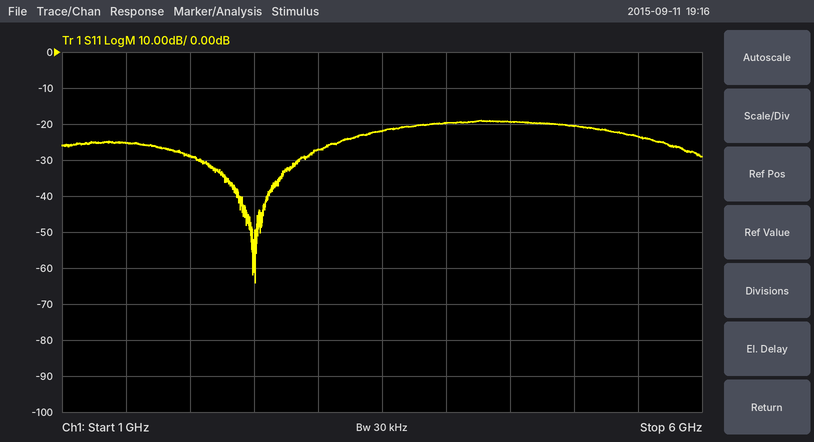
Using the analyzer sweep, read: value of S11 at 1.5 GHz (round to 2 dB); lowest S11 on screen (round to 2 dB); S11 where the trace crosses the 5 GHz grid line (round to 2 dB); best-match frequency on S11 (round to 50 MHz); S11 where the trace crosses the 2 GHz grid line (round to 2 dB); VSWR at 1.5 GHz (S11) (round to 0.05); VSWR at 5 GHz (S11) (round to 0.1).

-26 dB
-64 dB
-20 dB
2.50 GHz
-28 dB
1.10
1.2
